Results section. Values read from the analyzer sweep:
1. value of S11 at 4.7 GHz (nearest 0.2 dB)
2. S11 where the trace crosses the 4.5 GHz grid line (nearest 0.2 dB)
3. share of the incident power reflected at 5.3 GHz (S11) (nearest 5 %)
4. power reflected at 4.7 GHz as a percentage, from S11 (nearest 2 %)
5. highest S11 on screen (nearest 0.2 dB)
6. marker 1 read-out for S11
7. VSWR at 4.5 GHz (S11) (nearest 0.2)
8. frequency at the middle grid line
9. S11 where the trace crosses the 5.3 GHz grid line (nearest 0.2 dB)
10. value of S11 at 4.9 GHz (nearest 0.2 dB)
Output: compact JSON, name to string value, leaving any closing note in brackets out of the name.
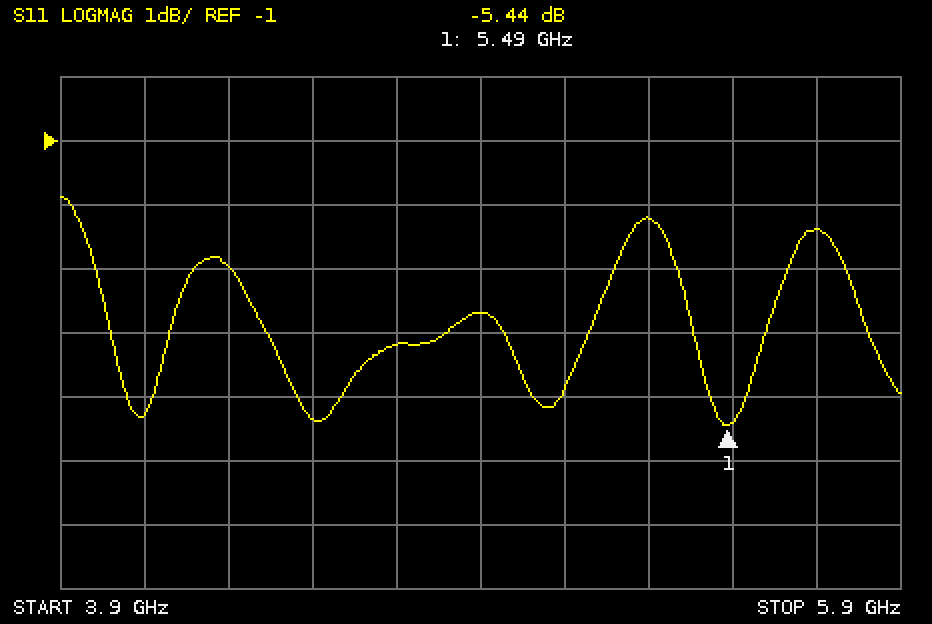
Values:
{"value of S11 at 4.7 GHz": "-4.2 dB", "S11 where the trace crosses the 4.5 GHz grid line": "-5.4 dB", "share of the incident power reflected at 5.3 GHz (S11)": "60 %", "power reflected at 4.7 GHz as a percentage, from S11": "38 %", "highest S11 on screen": "-1.8 dB", "marker 1 read-out for S11": "-5.44 dB", "VSWR at 4.5 GHz (S11)": "3.4", "frequency at the middle grid line": "4.9 GHz", "S11 where the trace crosses the 5.3 GHz grid line": "-2.2 dB", "value of S11 at 4.9 GHz": "-3.6 dB"}
